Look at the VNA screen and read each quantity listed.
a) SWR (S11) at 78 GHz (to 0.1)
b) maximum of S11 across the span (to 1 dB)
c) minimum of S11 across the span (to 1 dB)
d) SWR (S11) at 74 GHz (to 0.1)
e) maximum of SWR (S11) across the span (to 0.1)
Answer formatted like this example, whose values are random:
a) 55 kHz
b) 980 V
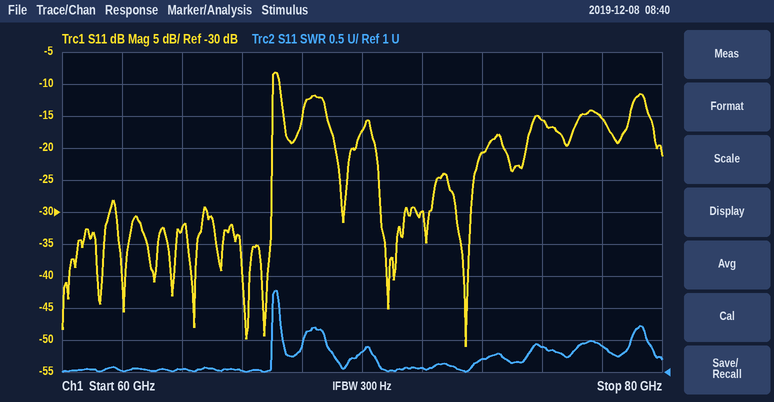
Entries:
a) 1.4
b) -8 dB
c) -51 dB
d) 1.2
e) 2.3
